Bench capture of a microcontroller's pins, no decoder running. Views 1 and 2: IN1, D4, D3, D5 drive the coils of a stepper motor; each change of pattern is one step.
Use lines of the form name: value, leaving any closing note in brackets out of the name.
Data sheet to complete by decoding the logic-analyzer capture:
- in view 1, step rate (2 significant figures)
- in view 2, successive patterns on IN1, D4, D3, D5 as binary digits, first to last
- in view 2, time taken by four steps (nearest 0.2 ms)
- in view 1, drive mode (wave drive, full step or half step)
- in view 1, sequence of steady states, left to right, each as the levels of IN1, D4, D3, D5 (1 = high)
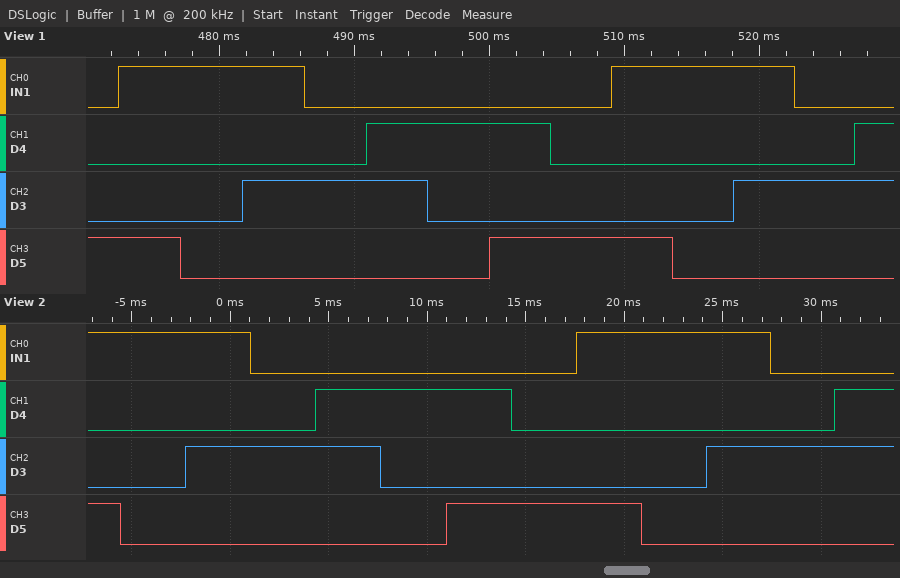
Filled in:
in view 1, step rate: 220 steps/s
in view 2, successive patterns on IN1, D4, D3, D5 as binary digits, first to last: 1001 1000 1010 0010 0110 0100 0101 0001 1001 1000 1010 0010 0110
in view 2, time taken by four steps: 13.2 ms
in view 1, drive mode: half step
in view 1, sequence of steady states, left to right, each as the levels of IN1, D4, D3, D5: 0001 1001 1000 1010 0010 0110 0100 0101 0001 1001 1000 1010 0010 0110
